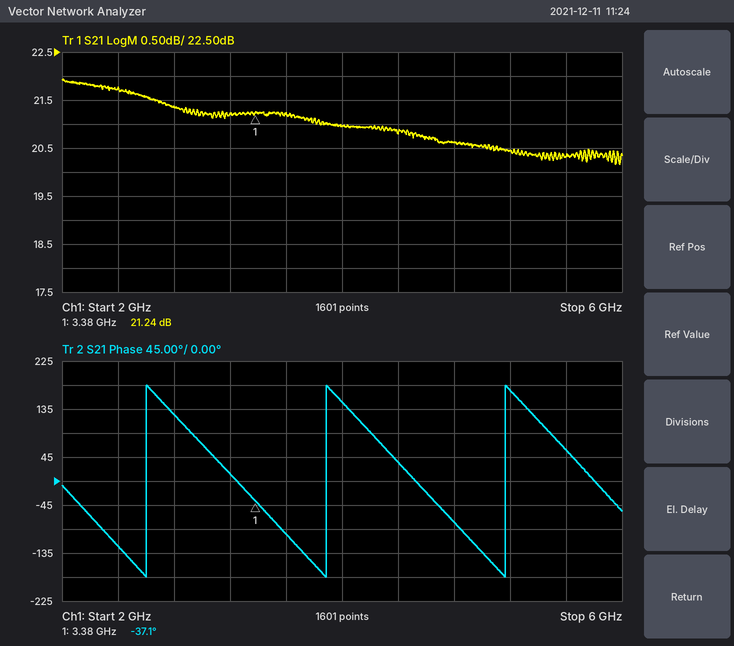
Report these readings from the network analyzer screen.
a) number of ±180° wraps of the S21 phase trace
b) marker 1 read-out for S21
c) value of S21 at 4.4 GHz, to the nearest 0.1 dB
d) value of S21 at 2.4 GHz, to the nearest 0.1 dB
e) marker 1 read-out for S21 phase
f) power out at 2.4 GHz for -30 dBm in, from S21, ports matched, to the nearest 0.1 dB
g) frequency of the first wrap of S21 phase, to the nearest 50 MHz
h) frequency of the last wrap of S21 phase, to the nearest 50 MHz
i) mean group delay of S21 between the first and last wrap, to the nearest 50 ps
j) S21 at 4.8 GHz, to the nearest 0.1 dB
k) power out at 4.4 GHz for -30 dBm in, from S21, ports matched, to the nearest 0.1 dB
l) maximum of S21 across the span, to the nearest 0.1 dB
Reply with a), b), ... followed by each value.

a) 3
b) 21.24 dB
c) 20.8 dB
d) 21.7 dB
e) -37.1°
f) -8.3 dBm
g) 2.60 GHz
h) 5.15 GHz
i) 800 ps
j) 20.6 dB
k) -9.2 dBm
l) 21.9 dB
